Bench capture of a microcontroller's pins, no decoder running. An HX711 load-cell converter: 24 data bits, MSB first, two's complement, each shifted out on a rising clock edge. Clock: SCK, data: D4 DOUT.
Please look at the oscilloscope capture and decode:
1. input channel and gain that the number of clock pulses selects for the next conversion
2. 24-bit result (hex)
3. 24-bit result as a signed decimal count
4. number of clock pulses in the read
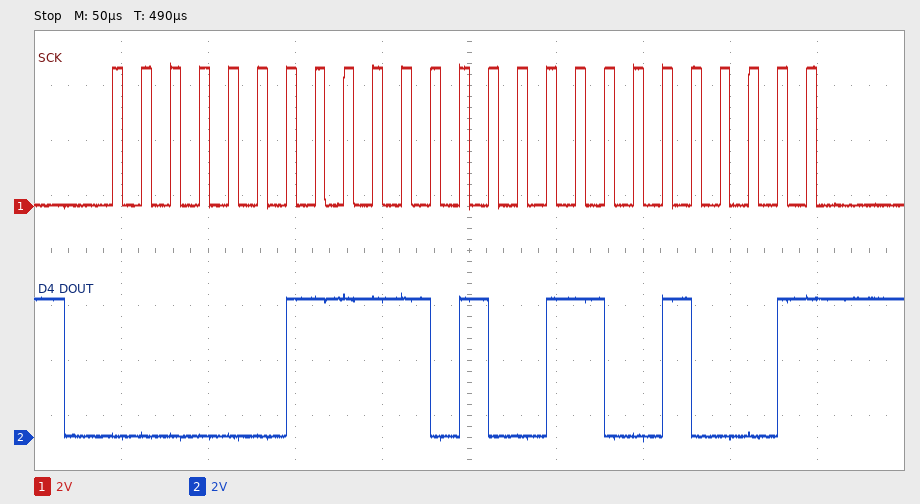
channel A, gain 128
0x03E991
256401
25
